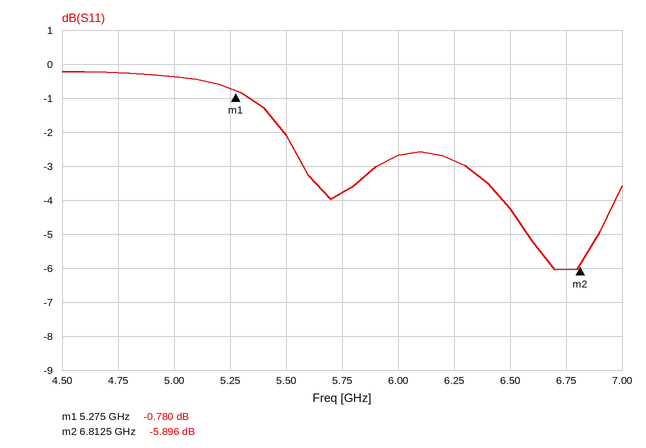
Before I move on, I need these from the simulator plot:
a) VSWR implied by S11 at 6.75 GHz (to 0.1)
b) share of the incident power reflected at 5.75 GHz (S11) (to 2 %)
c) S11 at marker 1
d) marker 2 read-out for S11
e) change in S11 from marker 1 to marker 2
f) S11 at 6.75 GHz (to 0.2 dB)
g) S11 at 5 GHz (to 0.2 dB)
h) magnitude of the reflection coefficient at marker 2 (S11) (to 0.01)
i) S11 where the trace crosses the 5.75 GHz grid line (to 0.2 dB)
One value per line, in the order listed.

3.0
42 %
-0.780 dB
-5.896 dB
-5.116 dB
-6.0 dB
-0.4 dB
0.51
-3.8 dB
